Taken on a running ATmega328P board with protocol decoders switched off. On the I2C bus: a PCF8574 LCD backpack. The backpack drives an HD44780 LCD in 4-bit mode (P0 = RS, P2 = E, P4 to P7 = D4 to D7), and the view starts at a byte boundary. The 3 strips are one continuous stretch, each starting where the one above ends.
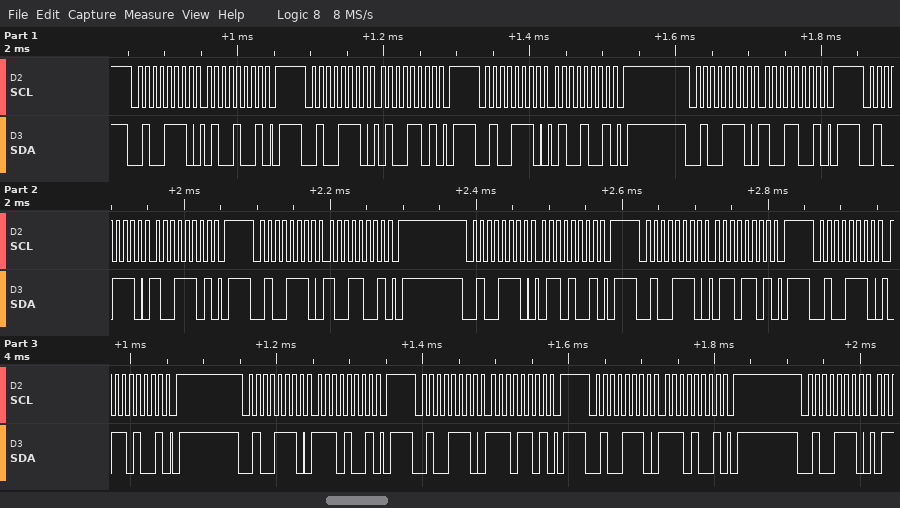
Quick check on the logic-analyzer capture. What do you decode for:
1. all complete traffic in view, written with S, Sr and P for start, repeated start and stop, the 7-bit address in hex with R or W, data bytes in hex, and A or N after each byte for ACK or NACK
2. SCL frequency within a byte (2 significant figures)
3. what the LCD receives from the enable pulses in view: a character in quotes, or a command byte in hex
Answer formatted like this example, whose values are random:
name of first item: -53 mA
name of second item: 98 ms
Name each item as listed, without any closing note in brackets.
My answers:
all complete traffic in view, written with S, Sr and P for start, repeated start and stop, the 7-bit address in hex with R or W, data bytes in hex, and A or N after each byte for ACK or NACK: S 27W A 49 A P S 27W A 4D A P S 27W A 49 A P S 27W A 99 A P S 27W A 9D A P S 27W A 99 A P S 27W A 69 A P S 27W A 6D A P S 27W A 69 A P S 27W A E9 A P S 27W A ED A P S 27W A E9 A P S 27W A
SCL frequency within a byte: 100 kHz
what the LCD receives from the enable pulses in view: a character in quotes, or a command byte in hex: 'I' 'n'
